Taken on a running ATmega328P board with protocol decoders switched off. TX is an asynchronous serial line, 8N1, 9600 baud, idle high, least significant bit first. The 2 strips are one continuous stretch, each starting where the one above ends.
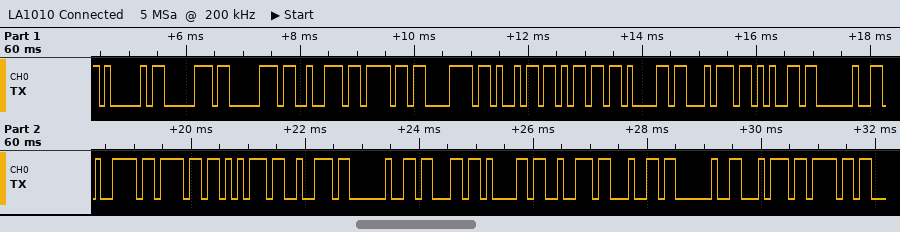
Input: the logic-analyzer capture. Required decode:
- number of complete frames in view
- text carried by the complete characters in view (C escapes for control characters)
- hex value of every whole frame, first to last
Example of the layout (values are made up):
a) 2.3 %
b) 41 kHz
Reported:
a) 24
b) "Approximate your card to"
c) 41 70 70 72 6F 78 69 6D 61 74 65 20 79 6F 75 72 20 63 61 72 64 20 74 6F
